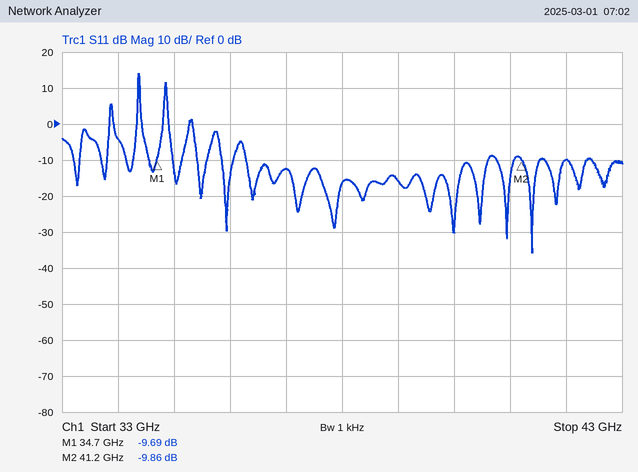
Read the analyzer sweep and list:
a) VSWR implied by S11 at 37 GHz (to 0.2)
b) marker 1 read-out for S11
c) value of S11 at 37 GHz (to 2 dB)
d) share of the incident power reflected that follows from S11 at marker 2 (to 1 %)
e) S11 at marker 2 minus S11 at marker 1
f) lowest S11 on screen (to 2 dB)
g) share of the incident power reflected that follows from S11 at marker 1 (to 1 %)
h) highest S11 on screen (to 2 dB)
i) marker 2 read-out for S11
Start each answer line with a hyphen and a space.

- 1.6
- -9.69 dB
- -12 dB
- 10 %
- -0.17 dB
- -36 dB
- 11 %
- 14 dB
- -9.86 dB
